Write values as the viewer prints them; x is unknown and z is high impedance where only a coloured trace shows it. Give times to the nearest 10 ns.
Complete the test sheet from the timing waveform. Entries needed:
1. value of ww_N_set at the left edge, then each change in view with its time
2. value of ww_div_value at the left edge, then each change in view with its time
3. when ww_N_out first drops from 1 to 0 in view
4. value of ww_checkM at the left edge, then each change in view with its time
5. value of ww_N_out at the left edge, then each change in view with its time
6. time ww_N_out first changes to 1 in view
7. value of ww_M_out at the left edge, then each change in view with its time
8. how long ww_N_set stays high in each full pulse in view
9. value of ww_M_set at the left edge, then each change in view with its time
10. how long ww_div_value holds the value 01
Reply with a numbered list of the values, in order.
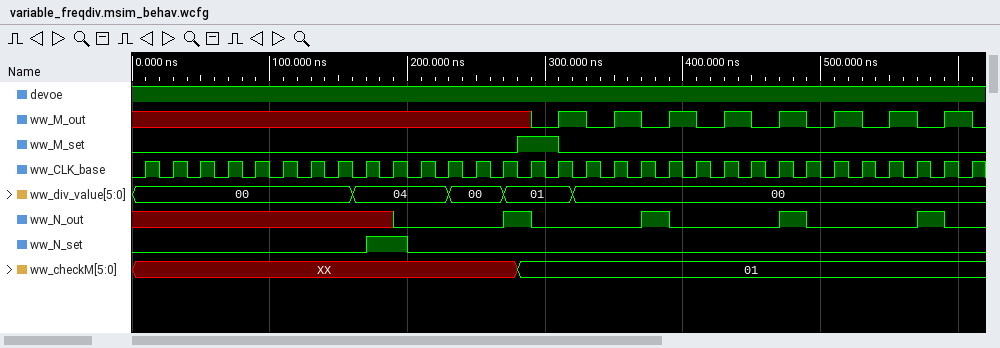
1. 0, 1 at 170 ns, 0 at 200 ns
2. 00, 04 at 160 ns, 00 at 230 ns, 01 at 270 ns, 00 at 320 ns
3. 290 ns
4. XX, 01 at 280 ns
5. x, 0 at 190 ns, 1 at 270 ns, 0 at 290 ns, 1 at 370 ns, 0 at 390 ns, 1 at 470 ns, 0 at 490 ns, 1 at 570 ns, 0 at 590 ns
6. 270 ns
7. x, 0 at 290 ns, 1 at 310 ns, 0 at 330 ns, 1 at 350 ns, 0 at 370 ns, 1 at 390 ns, 0 at 410 ns, 1 at 430 ns, 0 at 450 ns, 1 at 470 ns, 0 at 490 ns, 1 at 510 ns, 0 at 530 ns, 1 at 550 ns, 0 at 570 ns, 1 at 590 ns, 0 at 610 ns
8. 30 ns
9. 0, 1 at 280 ns, 0 at 310 ns
10. 50 ns
